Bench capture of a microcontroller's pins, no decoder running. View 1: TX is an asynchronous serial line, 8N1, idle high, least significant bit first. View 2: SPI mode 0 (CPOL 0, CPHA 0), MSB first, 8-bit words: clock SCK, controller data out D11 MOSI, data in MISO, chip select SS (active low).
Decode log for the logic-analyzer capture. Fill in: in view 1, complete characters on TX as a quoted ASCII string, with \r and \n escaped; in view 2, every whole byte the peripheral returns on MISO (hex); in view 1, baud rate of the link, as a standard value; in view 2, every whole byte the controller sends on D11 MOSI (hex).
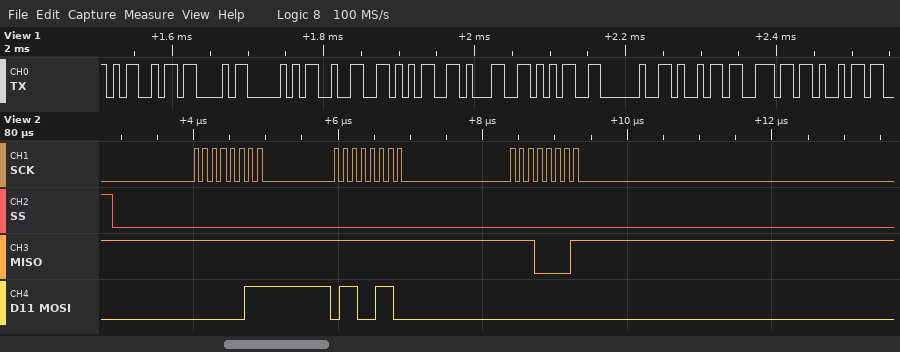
"MCP2515 ini"
FF FF E1
115200 baud
03 66 00
